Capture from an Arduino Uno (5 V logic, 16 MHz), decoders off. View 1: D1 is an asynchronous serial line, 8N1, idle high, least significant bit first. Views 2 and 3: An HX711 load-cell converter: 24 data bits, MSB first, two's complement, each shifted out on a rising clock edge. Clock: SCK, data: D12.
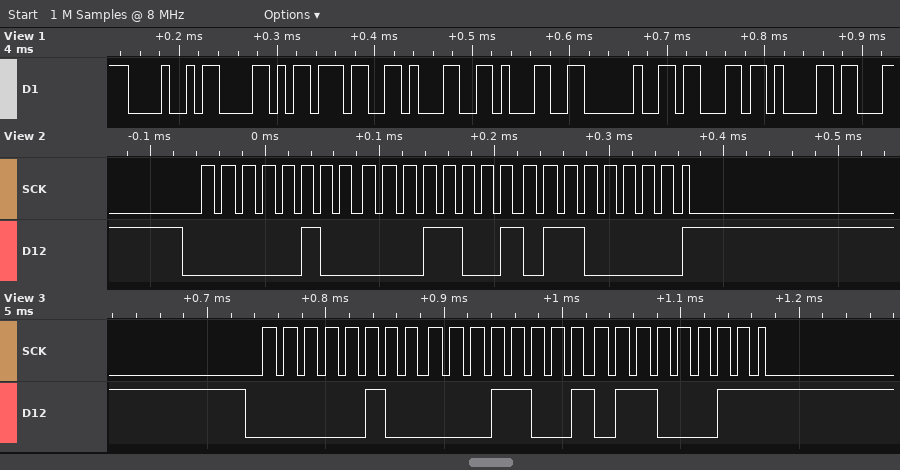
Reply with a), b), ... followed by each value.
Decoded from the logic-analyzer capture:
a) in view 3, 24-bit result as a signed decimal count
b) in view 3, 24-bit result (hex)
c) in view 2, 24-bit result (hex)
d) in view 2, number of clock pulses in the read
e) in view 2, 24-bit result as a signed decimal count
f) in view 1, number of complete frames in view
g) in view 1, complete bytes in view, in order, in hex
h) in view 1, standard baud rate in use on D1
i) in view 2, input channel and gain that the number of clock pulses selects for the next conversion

a) 268643
b) 0x041963
c) 0x041960
d) 25
e) 268640
f) 8
g) 0x48 0x58 0x37 0x31 0x31 0x20 0x63 0x61
h) 115200 baud
i) channel A, gain 128
